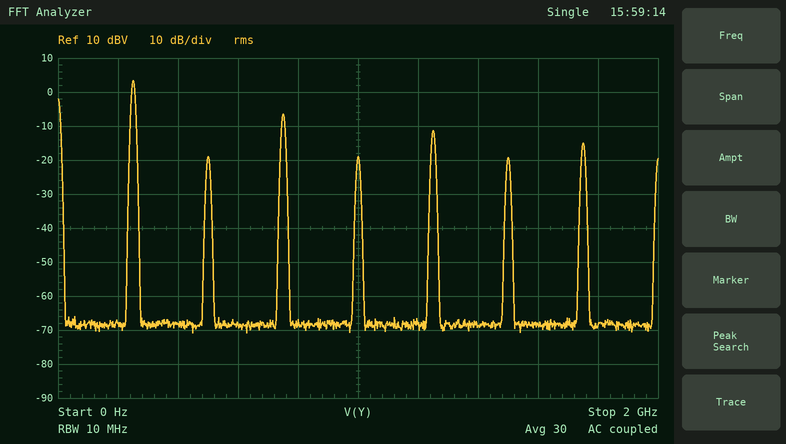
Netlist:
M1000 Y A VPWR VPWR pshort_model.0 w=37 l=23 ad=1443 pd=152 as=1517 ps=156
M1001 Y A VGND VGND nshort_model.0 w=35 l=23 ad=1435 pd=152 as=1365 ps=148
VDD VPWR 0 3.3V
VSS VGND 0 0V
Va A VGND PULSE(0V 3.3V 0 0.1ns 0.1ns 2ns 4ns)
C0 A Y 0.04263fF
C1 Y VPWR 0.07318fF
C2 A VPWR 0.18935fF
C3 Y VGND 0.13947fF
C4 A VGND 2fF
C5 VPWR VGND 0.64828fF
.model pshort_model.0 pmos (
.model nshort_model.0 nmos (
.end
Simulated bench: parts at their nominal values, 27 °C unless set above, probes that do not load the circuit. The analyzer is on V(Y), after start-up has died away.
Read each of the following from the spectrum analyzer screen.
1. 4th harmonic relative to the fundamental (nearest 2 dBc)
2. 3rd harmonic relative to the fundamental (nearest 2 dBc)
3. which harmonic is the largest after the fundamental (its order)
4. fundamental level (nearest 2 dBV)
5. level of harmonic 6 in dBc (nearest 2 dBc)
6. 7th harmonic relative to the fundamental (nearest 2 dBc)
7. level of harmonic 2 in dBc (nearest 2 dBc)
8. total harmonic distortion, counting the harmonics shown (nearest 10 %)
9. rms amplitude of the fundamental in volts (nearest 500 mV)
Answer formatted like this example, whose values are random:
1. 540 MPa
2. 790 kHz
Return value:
1. -22 dBc
2. -10 dBc
3. 3
4. 4 dBV
5. -22 dBc
6. -18 dBc
7. -22 dBc
8. 40 %
9. 1.5 V
